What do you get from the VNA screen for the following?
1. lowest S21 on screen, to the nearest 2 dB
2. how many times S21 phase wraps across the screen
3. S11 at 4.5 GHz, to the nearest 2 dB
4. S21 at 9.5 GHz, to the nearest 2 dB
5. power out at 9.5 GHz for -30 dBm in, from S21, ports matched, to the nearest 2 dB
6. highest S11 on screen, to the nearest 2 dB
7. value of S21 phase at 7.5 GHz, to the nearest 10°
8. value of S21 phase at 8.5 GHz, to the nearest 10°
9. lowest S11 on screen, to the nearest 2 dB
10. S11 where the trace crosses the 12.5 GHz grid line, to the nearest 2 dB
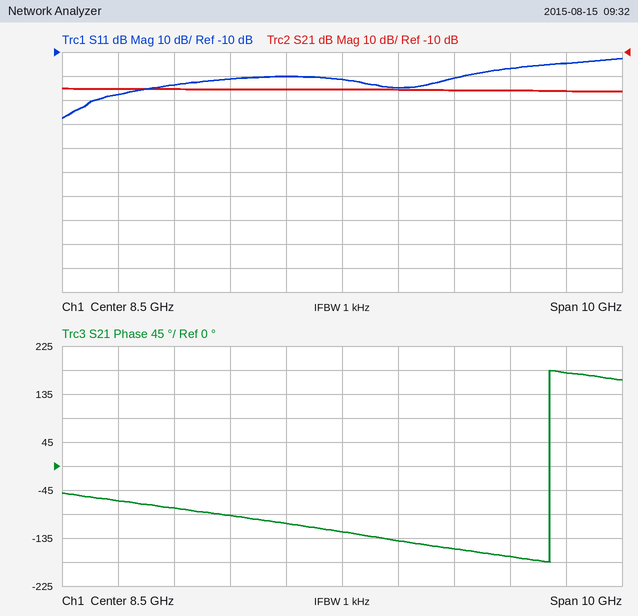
-26 dB
1
-28 dB
-26 dB
-56 dBm
-12 dB
-110°
-120°
-38 dB
-14 dB
